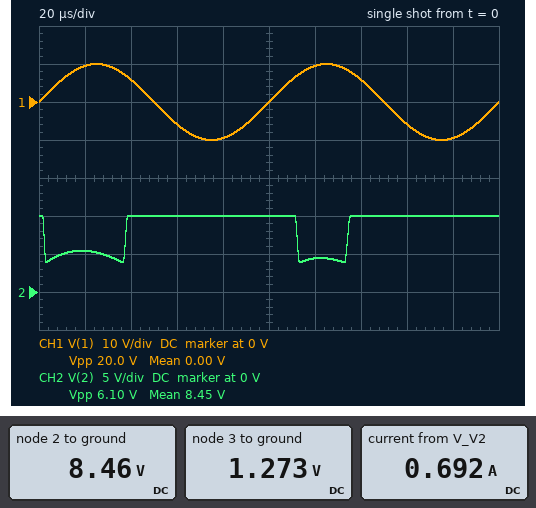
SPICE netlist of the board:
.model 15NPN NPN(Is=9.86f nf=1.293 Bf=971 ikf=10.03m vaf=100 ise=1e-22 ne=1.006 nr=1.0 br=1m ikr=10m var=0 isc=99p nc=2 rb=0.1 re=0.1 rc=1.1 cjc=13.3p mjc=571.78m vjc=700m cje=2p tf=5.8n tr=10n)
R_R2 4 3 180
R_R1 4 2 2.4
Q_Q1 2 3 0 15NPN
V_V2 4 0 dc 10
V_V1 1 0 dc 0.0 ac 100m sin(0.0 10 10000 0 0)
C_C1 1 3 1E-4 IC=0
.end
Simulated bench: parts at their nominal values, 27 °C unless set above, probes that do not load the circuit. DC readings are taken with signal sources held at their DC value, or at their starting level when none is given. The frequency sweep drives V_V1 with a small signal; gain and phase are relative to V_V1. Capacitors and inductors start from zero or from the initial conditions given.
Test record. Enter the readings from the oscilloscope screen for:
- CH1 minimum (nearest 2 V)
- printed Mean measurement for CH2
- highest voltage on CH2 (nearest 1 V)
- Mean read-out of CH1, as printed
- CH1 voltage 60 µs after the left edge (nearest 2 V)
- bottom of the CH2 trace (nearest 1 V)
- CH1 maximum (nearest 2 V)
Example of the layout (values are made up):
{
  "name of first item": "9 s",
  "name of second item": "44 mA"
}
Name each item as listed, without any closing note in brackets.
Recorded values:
{
  "CH1 minimum": "-10 V",
  "printed Mean measurement for CH2": "8.45 V",
  "highest voltage on CH2": "10 V",
  "Mean read-out of CH1, as printed": "0.00 V",
  "CH1 voltage 60 µs after the left edge": "-6 V",
  "bottom of the CH2 trace": "4 V",
  "CH1 maximum": "10 V"
}
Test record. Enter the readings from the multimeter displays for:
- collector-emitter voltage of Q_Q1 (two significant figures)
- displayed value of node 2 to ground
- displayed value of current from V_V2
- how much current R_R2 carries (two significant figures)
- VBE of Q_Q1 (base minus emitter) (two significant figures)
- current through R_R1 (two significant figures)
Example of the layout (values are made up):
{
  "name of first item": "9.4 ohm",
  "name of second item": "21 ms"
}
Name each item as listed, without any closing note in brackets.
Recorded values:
{
  "collector-emitter voltage of Q_Q1": "8.5 V",
  "displayed value of node 2 to ground": "8.46 V",
  "displayed value of current from V_V2": "0.692 A",
  "how much current R_R2 carries": "48 mA",
  "VBE of Q_Q1 (base minus emitter)": "1.3 V",
  "current through R_R1": "640 mA"
}
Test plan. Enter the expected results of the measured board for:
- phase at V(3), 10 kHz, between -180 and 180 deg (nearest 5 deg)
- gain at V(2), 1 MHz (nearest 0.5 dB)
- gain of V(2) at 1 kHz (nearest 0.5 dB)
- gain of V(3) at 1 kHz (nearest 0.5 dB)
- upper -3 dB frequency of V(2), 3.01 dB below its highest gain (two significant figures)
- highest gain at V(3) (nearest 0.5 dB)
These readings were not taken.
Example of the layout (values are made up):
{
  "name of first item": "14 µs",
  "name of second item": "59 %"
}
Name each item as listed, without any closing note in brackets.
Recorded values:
{
  "phase at V(3), 10 kHz, between -180 and 180 deg": "5 deg",
  "gain at V(2), 1 MHz": "20.0 dB",
  "gain of V(2) at 1 kHz": "16.5 dB",
  "gain of V(3) at 1 kHz": "-3.5 dB",
  "upper -3 dB frequency of V(2), 3.01 dB below its highest gain": "33 MHz",
  "highest gain at V(3)": "0 dB"
}
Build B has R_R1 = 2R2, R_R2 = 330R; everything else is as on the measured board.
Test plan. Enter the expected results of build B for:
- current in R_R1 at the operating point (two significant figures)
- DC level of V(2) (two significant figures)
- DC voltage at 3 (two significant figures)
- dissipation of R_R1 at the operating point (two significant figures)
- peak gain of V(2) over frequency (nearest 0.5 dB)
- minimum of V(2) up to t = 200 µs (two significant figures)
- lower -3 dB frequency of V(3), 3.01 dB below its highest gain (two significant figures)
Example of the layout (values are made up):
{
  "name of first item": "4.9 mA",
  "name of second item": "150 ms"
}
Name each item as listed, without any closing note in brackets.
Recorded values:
{
  "current in R_R1 at the operating point": "490 mA",
  "DC level of V(2)": "8.9 V",
  "DC voltage at 3": "1.2 V",
  "dissipation of R_R1 at the operating point": "520 mW",
  "peak gain of V(2) over frequency": "18.5 dB",
  "minimum of V(2) up to t = 200 µs": "4.1 V",
  "lower -3 dB frequency of V(3), 3.01 dB below its highest gain": "710 Hz"
}
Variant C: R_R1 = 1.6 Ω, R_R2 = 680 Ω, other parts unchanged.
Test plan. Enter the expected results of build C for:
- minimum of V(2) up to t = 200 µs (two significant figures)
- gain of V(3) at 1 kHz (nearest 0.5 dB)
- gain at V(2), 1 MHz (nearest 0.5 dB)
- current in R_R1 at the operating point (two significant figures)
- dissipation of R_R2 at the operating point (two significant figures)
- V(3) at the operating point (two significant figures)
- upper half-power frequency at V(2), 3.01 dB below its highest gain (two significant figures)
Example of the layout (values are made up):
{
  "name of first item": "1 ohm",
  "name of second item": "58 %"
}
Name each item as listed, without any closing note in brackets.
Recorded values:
{
  "minimum of V(2) up to t = 200 µs": "4.8 V",
  "gain of V(3) at 1 kHz": "-0.5 dB",
  "gain at V(2), 1 MHz": "14.5 dB",
  "current in R_R1 at the operating point": "350 mA",
  "dissipation of R_R2 at the operating point": "110 mW",
  "V(3) at the operating point": "1.2 V",
  "upper half-power frequency at V(2), 3.01 dB below its highest gain": "42 MHz"
}
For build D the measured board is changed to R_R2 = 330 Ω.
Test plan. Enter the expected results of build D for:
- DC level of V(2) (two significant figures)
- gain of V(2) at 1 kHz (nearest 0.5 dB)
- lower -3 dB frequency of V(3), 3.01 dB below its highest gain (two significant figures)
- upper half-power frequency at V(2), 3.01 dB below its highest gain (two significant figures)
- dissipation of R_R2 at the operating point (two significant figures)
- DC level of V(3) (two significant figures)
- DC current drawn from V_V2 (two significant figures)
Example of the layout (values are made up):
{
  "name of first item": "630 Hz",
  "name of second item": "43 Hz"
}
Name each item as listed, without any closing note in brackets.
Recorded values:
{
  "DC level of V(2)": "8.8 V",
  "gain of V(2) at 1 kHz": "17.5 dB",
  "lower -3 dB frequency of V(3), 3.01 dB below its highest gain": "710 Hz",
  "upper half-power frequency at V(2), 3.01 dB below its highest gain": "36 MHz",
  "dissipation of R_R2 at the operating point": "230 mW",
  "DC level of V(3)": "1.2 V",
  "DC current drawn from V_V2": "510 mA"
}
